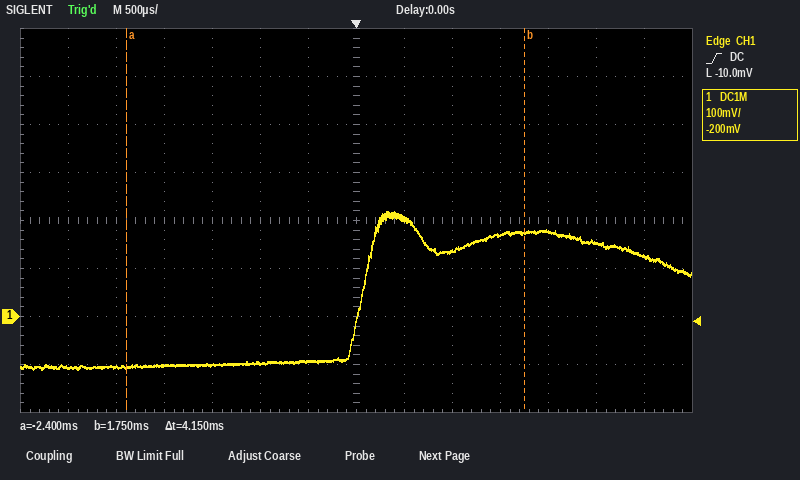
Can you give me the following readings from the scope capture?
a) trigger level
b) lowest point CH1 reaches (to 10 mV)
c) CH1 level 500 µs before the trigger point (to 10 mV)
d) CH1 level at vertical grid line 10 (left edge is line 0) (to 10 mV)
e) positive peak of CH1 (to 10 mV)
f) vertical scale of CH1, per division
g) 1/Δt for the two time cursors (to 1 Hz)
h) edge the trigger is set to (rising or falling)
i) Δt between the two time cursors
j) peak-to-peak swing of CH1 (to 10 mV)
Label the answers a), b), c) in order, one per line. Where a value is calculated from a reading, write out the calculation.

a) -10.0 mV
b) -110 mV
c) -90 mV
d) 170 mV
e) 220 mV
f) 100 mV
g) 1 / 4.15 ms ≈ 241 Hz
h) rising
i) 4.15 ms
j) 220 mV − (-110 mV) = 330 mV
